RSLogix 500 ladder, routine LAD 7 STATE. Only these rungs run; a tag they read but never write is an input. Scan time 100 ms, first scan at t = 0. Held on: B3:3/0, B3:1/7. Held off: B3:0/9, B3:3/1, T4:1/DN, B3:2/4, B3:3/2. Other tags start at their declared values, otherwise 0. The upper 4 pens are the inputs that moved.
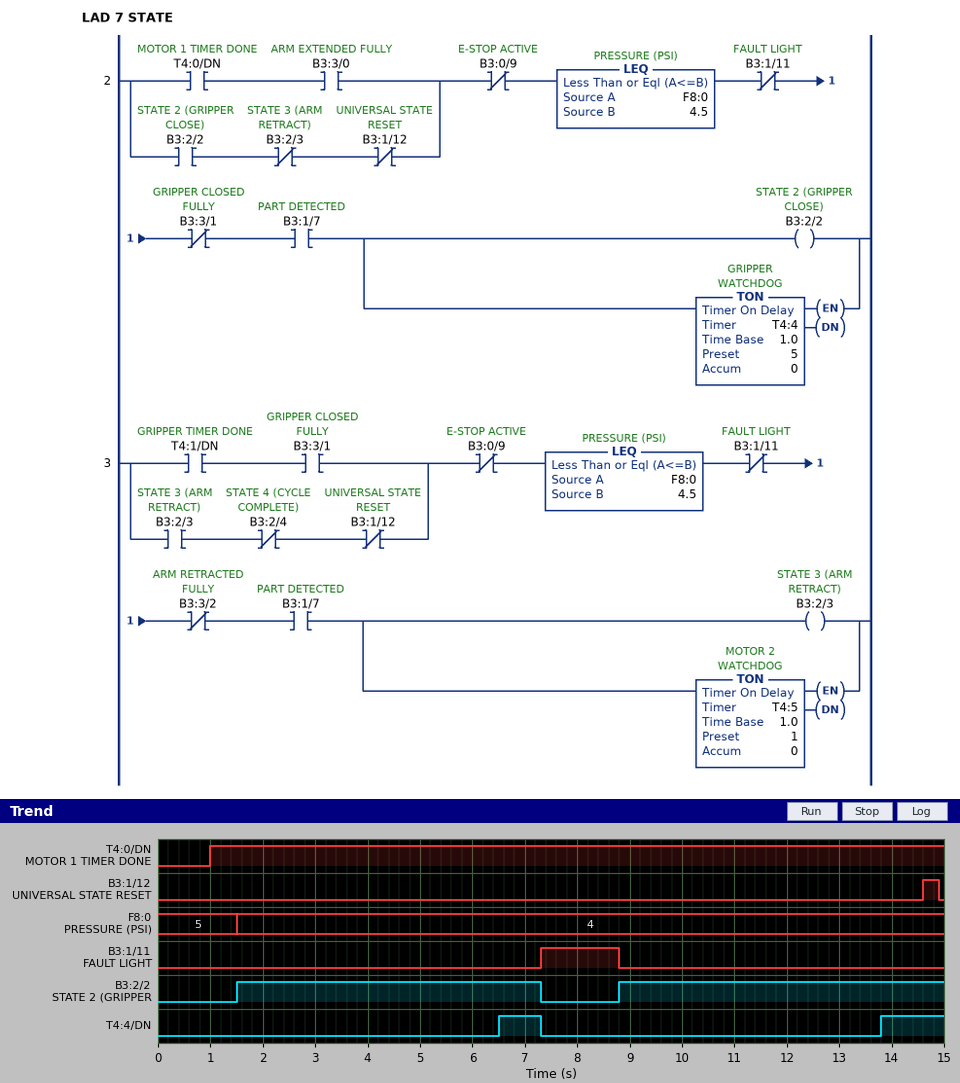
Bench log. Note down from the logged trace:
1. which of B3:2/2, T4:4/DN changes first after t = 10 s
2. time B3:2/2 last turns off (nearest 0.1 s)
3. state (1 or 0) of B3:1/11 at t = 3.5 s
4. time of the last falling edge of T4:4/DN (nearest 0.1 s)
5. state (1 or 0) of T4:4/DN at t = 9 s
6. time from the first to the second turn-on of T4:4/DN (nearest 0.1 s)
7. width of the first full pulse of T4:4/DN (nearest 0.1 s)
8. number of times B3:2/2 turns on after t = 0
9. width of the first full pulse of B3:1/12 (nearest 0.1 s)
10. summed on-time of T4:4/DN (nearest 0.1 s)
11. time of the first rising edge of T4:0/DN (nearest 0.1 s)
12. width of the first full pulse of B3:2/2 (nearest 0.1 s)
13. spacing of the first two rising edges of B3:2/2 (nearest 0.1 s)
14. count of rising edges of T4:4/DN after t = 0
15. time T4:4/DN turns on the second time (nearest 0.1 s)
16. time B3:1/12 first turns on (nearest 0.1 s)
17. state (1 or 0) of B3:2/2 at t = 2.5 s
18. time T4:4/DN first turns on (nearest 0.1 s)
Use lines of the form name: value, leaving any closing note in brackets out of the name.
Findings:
which of B3:2/2, T4:4/DN changes first after t = 10 s: T4:4/DN
time B3:2/2 last turns off: 7.3 s
state (1 or 0) of B3:1/11 at t = 3.5 s: 0
time of the last falling edge of T4:4/DN: 7.3 s
state (1 or 0) of T4:4/DN at t = 9 s: 0
time from the first to the second turn-on of T4:4/DN: 7.3 s
width of the first full pulse of T4:4/DN: 0.8 s
number of times B3:2/2 turns on after t = 0: 2
width of the first full pulse of B3:1/12: 0.3 s
summed on-time of T4:4/DN: 2.0 s
time of the first rising edge of T4:0/DN: 1.0 s
width of the first full pulse of B3:2/2: 5.8 s
spacing of the first two rising edges of B3:2/2: 7.3 s
count of rising edges of T4:4/DN after t = 0: 2
time T4:4/DN turns on the second time: 13.8 s
time B3:1/12 first turns on: 14.6 s
state (1 or 0) of B3:2/2 at t = 2.5 s: 1
time T4:4/DN first turns on: 6.5 s
